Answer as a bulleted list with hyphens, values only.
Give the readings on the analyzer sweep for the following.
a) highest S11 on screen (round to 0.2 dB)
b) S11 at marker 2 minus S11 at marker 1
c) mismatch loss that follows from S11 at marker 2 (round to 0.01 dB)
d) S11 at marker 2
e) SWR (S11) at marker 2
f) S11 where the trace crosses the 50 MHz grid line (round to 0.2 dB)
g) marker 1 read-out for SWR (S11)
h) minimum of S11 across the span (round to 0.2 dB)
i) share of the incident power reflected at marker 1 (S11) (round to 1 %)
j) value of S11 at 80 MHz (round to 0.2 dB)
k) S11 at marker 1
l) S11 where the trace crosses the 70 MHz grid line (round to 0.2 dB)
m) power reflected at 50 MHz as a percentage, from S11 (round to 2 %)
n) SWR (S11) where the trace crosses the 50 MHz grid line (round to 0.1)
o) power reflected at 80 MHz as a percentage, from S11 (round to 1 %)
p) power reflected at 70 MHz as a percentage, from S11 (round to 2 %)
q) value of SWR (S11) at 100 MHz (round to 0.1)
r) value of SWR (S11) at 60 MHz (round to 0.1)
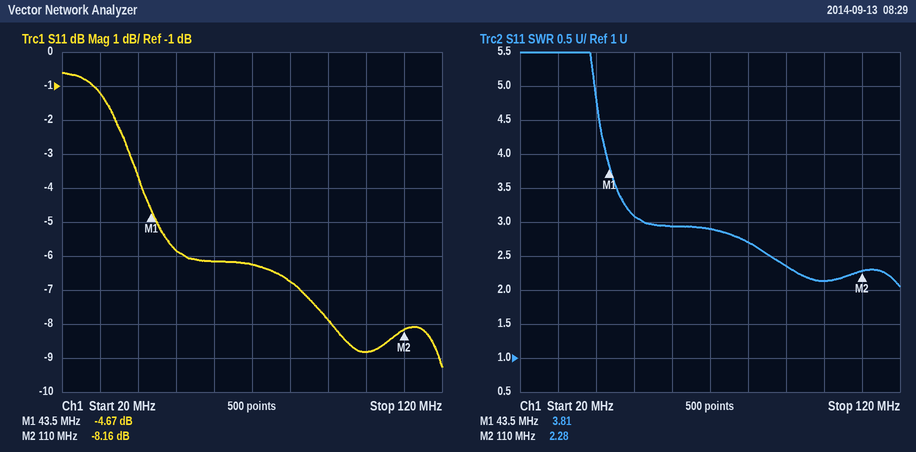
- -0.6 dB
- -3.49 dB
- 0.72 dB
- -8.16 dB
- 2.28
- -5.8 dB
- 3.81
- -9.2 dB
- 34 %
- -6.8 dB
- -4.67 dB
- -6.2 dB
- 26 %
- 3.1
- 21 %
- 24 %
- 2.1
- 2.9
